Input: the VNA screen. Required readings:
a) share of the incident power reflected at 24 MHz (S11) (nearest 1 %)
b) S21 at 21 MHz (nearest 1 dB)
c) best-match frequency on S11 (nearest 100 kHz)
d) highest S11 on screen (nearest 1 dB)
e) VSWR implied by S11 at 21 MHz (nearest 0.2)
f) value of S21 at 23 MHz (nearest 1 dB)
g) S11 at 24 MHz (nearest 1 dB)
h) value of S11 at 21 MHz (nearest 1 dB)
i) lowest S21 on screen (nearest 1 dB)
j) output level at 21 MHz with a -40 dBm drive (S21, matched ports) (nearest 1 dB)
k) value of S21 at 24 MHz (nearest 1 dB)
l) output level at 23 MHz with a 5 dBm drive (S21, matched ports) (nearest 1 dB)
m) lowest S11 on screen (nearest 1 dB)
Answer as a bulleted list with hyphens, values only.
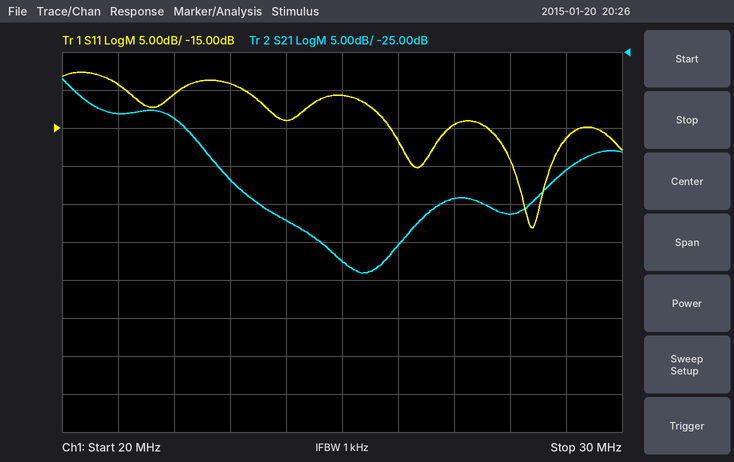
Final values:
- 4 %
- -33 dB
- 28.4 MHz
- -8 dB
- 2.0
- -42 dB
- -14 dB
- -9 dB
- -54 dB
- -73 dBm
- -47 dB
- -37 dBm
- -28 dB
